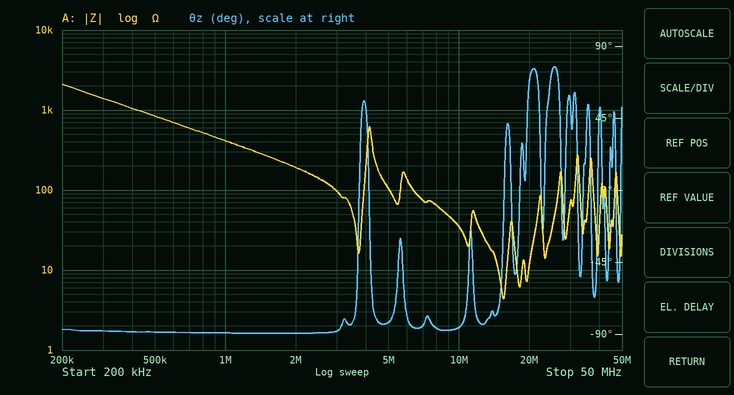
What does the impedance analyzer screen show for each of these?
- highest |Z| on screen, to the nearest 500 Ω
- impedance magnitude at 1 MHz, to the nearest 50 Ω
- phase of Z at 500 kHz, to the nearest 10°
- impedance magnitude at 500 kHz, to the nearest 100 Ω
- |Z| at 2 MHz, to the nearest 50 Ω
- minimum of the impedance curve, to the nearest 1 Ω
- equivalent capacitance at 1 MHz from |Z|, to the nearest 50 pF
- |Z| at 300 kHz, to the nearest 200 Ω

2.0 kΩ
400 Ω
-90°
800 Ω
200 Ω
4 Ω
400 pF
1.4 kΩ
